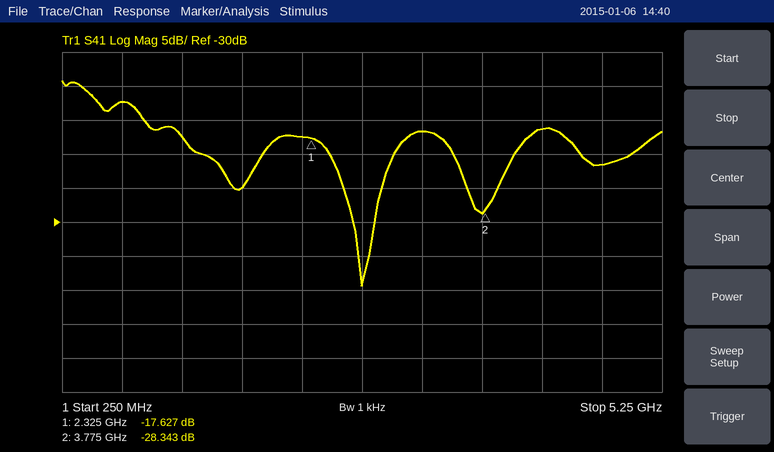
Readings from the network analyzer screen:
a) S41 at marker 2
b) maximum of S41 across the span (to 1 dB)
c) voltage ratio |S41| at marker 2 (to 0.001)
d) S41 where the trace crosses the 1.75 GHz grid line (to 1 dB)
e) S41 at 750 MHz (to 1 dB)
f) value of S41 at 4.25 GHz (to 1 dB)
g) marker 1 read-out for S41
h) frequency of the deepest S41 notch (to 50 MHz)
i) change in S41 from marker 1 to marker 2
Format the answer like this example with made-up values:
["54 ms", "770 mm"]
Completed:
["-28.343 dB", "-9 dB", "0.038", "-25 dB", "-12 dB", "-16 dB", "-17.627 dB", "2.75 GHz", "-10.716 dB"]
